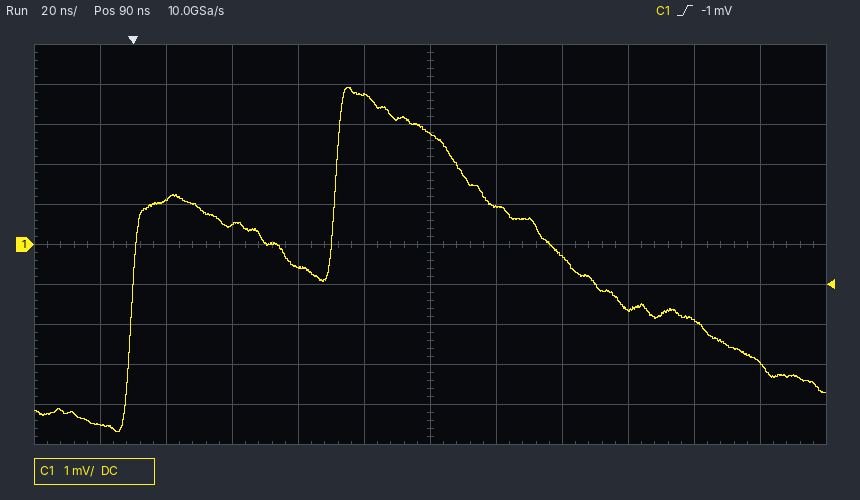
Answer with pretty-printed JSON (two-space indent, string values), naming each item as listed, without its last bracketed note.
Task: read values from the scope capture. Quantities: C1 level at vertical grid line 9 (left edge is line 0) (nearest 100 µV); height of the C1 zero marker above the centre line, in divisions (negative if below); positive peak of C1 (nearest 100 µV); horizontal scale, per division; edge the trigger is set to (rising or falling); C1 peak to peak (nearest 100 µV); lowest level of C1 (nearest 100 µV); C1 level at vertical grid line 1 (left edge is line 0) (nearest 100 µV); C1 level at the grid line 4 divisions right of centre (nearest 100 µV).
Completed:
{
  "C1 level at vertical grid line 9 (left edge is line 0)": "-1.6 mV",
  "height of the C1 zero marker above the centre line, in divisions": "0.0 div",
  "positive peak of C1": "3.9 mV",
  "horizontal scale, per division": "20 ns",
  "edge the trigger is set to": "rising",
  "C1 peak to peak": "8.6 mV",
  "lowest level of C1": "-4.7 mV",
  "C1 level at vertical grid line 1 (left edge is line 0)": "-4.5 mV",
  "C1 level at the grid line 4 divisions right of centre": "-1.9 mV"
}
